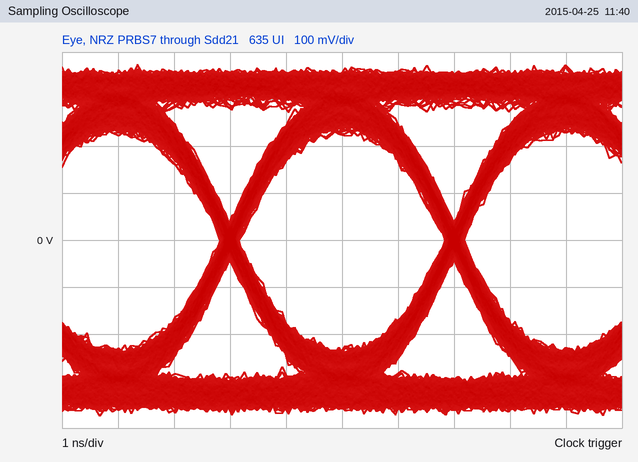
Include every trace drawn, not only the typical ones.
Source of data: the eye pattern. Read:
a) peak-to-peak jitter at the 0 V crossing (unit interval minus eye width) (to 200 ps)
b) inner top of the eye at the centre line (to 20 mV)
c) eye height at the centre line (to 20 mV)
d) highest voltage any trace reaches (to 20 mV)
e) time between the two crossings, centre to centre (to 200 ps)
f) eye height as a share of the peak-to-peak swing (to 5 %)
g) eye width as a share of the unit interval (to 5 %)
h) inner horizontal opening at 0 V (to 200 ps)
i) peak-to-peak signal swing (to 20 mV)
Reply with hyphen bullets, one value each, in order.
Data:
- 400 ps
- 220 mV
- 460 mV
- 380 mV
- 4.0 ns
- 60 %
- 90 %
- 3.6 ns
- 740 mV
